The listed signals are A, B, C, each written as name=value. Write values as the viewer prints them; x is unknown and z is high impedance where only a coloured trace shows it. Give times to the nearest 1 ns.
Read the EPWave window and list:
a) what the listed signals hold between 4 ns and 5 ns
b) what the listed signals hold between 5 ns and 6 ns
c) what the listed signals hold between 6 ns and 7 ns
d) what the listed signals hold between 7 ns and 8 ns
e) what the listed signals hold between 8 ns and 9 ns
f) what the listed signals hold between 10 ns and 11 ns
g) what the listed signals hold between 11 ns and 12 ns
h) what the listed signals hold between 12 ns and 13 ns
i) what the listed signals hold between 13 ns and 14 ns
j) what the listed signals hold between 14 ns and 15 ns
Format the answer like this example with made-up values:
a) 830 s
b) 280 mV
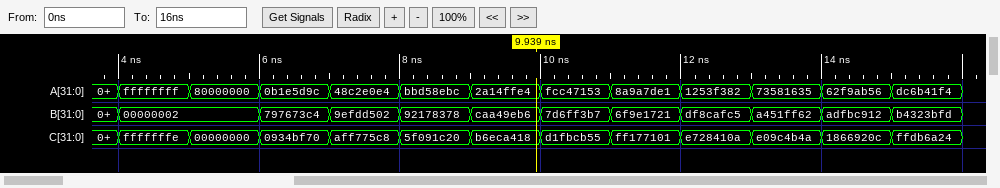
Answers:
a) A=ffffffff, B=00000002, C=fffffffe
b) A=80000000, B=00000002, C=00000000
c) A=0b1e5d9c, B=797673c4, C=0934bf70
d) A=48c2e0e4, B=9efdd502, C=aff775c8
e) A=bbd58ebc, B=92178378, C=5f091c20
f) A=fcc47153, B=7d6ff3b7, C=d1fbcb55
g) A=8a9a7de1, B=6f9e1721, C=ff177101
h) A=1253f382, B=df8cafc5, C=e728410a
i) A=73581635, B=a451ff62, C=e09c4b4a
j) A=62f9ab56, B=adfbc912, C=1866920c
